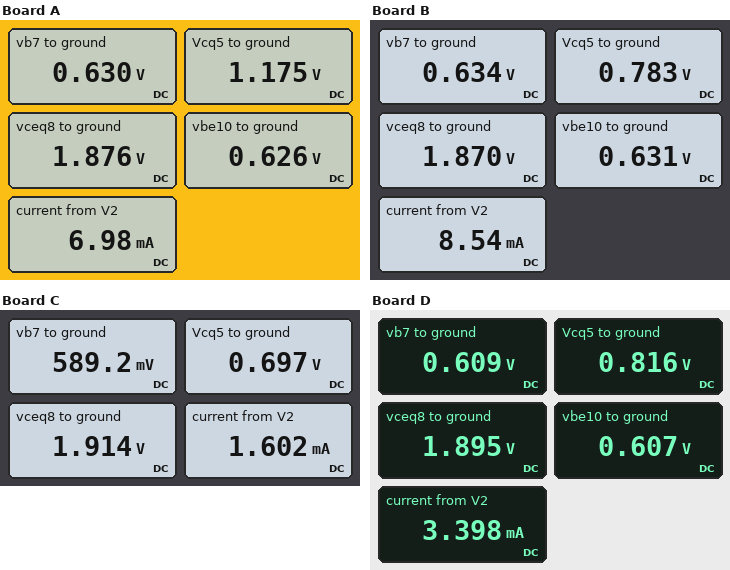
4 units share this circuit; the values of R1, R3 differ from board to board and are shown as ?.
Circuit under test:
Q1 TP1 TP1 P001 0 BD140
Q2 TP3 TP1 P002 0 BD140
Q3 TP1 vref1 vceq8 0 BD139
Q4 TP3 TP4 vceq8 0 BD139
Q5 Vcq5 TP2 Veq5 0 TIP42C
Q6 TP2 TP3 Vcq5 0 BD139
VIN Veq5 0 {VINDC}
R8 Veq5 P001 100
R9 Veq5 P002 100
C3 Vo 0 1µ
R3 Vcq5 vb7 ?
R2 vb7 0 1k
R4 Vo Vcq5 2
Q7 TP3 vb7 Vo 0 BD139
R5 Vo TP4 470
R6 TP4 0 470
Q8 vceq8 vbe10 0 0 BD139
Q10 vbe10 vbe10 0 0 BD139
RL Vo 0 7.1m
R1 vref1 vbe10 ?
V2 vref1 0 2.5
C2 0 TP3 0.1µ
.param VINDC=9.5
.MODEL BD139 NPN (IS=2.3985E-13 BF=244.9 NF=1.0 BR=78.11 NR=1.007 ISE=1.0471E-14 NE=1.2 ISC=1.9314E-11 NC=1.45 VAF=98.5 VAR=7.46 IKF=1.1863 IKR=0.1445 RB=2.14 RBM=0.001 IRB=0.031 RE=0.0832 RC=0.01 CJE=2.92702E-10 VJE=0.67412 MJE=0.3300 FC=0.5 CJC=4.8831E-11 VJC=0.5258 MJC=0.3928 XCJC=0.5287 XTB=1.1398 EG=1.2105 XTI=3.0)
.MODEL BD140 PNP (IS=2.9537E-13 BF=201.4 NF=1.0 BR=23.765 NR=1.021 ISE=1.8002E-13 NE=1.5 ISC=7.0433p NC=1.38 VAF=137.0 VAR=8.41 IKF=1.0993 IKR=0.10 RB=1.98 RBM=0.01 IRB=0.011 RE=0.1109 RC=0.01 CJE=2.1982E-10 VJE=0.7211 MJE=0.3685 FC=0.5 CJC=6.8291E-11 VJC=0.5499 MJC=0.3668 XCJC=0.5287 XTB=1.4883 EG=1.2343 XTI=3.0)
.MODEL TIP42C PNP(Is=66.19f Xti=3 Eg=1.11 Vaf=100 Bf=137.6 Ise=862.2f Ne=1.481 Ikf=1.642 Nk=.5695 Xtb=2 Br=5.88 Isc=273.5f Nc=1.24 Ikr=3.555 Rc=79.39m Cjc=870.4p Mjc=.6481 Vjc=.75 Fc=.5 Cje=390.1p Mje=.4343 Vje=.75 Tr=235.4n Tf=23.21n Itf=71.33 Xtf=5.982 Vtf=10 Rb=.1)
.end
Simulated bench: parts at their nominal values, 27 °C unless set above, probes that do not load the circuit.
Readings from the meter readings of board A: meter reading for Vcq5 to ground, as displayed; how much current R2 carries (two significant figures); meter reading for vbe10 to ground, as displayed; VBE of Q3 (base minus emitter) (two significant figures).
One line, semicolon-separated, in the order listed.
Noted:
1.175 V; 630 µA; 0.626 V; 620 mV
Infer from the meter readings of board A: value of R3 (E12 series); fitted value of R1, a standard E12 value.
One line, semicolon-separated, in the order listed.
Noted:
820 Ω; 270 Ω
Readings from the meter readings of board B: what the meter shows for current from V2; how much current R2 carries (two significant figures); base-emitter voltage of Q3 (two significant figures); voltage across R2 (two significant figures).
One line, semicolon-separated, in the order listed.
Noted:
8.54 mA; 630 µA; 630 mV; 630 mV
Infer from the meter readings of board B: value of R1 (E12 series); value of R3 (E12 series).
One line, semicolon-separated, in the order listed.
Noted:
220 Ω; 220 Ω
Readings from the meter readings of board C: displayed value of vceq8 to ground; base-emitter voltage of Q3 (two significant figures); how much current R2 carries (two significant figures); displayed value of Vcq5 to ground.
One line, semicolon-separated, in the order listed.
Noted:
1.914 V; 590 mV; 590 µA; 0.697 V
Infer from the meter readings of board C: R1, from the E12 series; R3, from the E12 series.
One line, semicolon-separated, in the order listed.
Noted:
1.2 kΩ; 180 Ω
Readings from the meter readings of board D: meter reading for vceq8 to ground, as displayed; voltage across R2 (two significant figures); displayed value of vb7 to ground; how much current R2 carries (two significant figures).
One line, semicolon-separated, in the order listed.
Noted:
1.895 V; 610 mV; 0.609 V; 610 µA
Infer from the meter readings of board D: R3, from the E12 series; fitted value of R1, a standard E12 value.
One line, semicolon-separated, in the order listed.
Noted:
330 Ω; 560 Ω
